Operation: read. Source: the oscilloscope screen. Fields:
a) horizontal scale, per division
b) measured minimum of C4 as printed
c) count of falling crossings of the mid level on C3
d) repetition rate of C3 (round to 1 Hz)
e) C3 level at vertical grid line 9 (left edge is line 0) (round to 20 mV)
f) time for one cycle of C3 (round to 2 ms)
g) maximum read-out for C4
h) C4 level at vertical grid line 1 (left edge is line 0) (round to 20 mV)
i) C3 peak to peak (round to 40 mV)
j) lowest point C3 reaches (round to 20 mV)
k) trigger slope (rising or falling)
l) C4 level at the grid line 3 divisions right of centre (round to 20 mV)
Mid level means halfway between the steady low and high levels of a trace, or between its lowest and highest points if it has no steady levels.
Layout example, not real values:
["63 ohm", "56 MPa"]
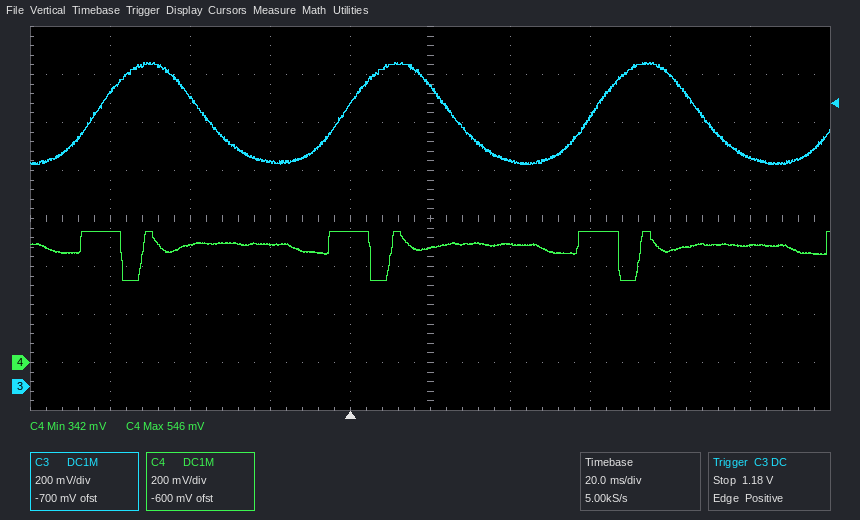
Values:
["20 ms", "342 mV", "3", "16 Hz", "960 mV", "62 ms", "546 mV", "540 mV", "440 mV", "920 mV", "rising", "460 mV"]
